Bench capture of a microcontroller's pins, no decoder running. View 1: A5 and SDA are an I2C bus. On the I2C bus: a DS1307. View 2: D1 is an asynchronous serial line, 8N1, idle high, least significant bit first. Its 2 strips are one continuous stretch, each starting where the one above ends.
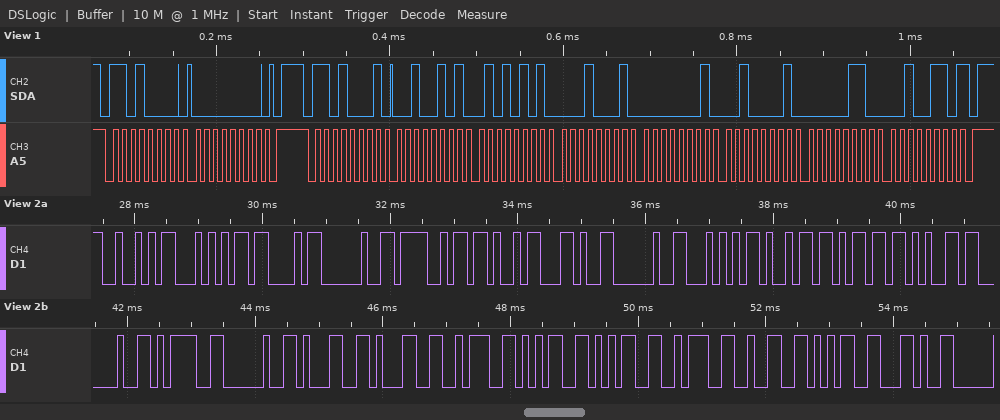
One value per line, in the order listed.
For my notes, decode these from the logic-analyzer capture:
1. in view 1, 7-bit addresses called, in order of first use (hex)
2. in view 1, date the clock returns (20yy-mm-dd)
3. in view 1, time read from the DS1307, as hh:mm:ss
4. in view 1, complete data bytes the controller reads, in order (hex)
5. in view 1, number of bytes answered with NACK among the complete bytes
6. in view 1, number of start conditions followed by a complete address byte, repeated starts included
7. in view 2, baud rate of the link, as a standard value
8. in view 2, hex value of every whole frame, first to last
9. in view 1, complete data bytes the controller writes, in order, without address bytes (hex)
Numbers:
0x68
2026-06-21
11:55:25
25 55 11 01 21 06 26
1
2
9600 baud
52 54 43 20 4F 4B 2C 20 54 69 6D 65 20 3D 20 31 31 3A 35 35 3A 32 35 2C
00
